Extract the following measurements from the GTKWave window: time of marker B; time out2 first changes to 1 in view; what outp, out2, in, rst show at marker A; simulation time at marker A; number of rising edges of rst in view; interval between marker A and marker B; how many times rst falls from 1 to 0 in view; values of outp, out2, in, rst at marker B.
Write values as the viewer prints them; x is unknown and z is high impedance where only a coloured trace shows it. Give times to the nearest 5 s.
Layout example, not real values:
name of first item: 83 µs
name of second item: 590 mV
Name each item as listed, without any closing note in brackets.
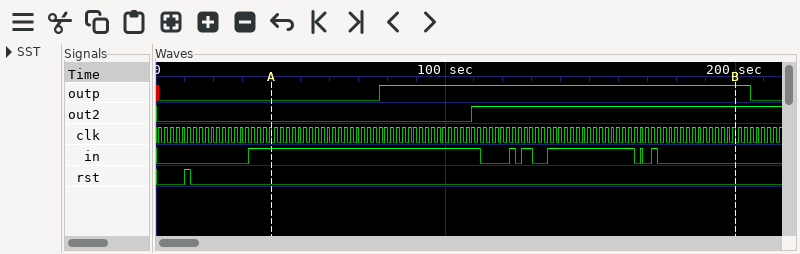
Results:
time of marker B: 200 s
time out2 first changes to 1 in view: 110 s
what outp, out2, in, rst show at marker A: outp=0, out2=0, in=1, rst=0
simulation time at marker A: 40 s
number of rising edges of rst in view: 1
interval between marker A and marker B: 160 s
how many times rst falls from 1 to 0 in view: 1
values of outp, out2, in, rst at marker B: outp=1, out2=1, in=0, rst=0
